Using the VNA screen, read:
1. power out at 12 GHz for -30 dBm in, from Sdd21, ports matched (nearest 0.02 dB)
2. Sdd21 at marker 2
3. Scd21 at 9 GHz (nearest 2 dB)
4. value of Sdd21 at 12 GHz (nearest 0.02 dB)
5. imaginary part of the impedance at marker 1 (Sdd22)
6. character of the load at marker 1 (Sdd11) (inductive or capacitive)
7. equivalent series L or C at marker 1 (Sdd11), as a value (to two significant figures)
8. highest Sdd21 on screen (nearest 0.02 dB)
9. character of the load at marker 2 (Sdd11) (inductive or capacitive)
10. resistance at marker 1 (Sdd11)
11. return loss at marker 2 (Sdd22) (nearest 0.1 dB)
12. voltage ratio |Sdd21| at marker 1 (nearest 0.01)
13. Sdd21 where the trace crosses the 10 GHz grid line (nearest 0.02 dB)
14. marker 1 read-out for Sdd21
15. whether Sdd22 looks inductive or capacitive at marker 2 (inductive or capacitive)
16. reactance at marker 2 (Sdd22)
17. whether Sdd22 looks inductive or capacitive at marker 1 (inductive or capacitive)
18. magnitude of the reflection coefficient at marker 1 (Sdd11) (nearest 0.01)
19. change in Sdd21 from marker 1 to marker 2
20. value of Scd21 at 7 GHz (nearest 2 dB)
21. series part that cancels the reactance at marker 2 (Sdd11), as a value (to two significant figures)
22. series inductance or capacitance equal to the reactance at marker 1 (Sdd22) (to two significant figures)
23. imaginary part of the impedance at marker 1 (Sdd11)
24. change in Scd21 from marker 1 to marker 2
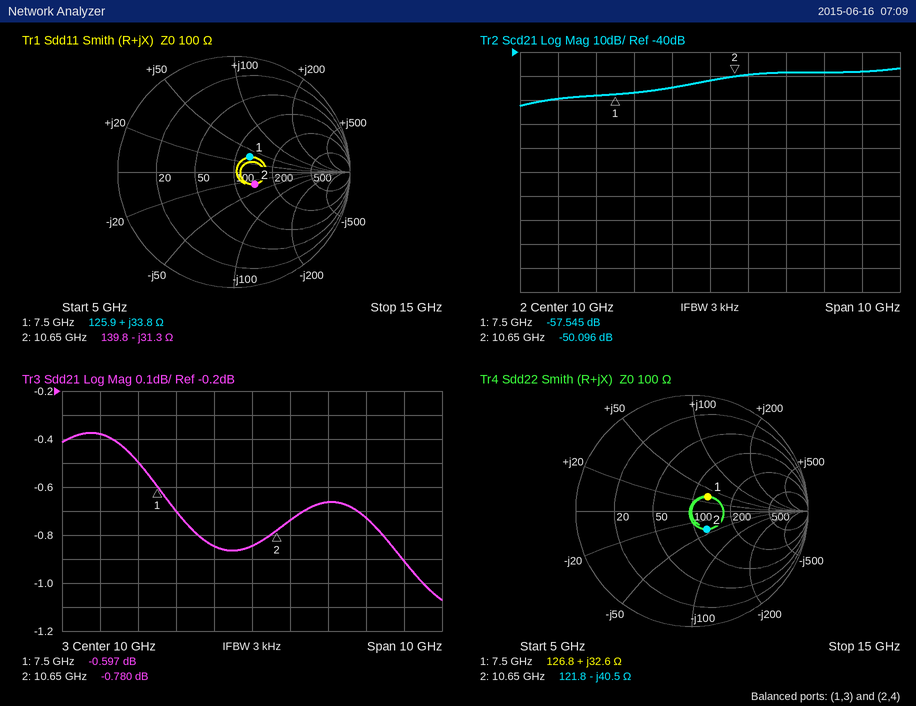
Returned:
-30.66 dBm
-0.780 dB
-54 dB
-0.66 dB
+32.6 Ω
inductive
720 pH
-0.38 dB
capacitive
125.9 Ω
13.8 dB
0.93
-0.84 dB
-0.597 dB
capacitive
-40.5 Ω
inductive
0.19
-0.183 dB
-58 dB
470 pH
690 pH
+33.8 Ω
7.449 dB
